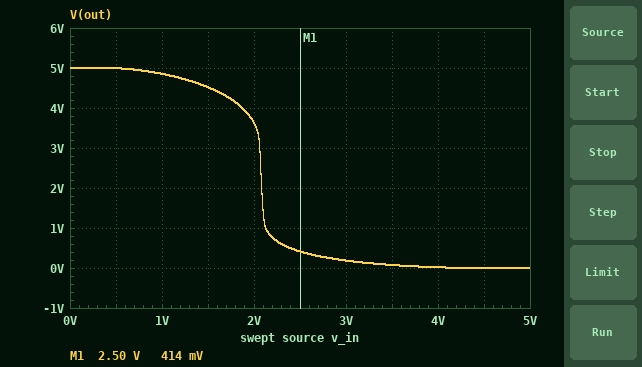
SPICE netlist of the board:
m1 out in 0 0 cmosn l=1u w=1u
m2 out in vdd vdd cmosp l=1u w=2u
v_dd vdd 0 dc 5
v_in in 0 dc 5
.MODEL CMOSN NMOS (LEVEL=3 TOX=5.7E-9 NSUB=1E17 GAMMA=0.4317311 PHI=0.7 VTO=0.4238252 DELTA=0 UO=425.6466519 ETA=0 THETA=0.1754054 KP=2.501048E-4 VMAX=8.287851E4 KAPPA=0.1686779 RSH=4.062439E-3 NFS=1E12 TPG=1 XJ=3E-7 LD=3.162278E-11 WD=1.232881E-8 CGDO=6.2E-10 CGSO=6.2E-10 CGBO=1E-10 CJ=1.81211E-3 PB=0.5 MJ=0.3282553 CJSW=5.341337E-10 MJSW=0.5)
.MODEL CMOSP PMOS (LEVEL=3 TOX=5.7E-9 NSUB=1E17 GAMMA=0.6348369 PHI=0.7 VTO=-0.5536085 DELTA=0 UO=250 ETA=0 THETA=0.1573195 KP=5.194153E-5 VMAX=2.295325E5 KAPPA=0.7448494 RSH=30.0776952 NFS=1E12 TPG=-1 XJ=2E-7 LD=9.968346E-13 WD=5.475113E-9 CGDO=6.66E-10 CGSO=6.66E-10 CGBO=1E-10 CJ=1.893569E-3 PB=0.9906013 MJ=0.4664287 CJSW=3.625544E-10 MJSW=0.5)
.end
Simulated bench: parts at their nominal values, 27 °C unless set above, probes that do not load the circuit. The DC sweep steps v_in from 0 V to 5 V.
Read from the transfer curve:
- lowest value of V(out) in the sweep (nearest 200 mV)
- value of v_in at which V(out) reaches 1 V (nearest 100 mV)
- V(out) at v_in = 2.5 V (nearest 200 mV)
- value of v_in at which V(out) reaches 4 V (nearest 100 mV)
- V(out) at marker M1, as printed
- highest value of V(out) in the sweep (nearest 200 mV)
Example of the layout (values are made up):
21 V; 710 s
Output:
0 V; 2.1 V; 400 mV; 1.9 V; 414 mV; 5.0 V
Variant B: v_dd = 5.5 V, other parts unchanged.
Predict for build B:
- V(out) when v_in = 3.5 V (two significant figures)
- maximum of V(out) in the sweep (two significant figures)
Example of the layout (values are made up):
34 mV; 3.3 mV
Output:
160 mV; 5.5 V
